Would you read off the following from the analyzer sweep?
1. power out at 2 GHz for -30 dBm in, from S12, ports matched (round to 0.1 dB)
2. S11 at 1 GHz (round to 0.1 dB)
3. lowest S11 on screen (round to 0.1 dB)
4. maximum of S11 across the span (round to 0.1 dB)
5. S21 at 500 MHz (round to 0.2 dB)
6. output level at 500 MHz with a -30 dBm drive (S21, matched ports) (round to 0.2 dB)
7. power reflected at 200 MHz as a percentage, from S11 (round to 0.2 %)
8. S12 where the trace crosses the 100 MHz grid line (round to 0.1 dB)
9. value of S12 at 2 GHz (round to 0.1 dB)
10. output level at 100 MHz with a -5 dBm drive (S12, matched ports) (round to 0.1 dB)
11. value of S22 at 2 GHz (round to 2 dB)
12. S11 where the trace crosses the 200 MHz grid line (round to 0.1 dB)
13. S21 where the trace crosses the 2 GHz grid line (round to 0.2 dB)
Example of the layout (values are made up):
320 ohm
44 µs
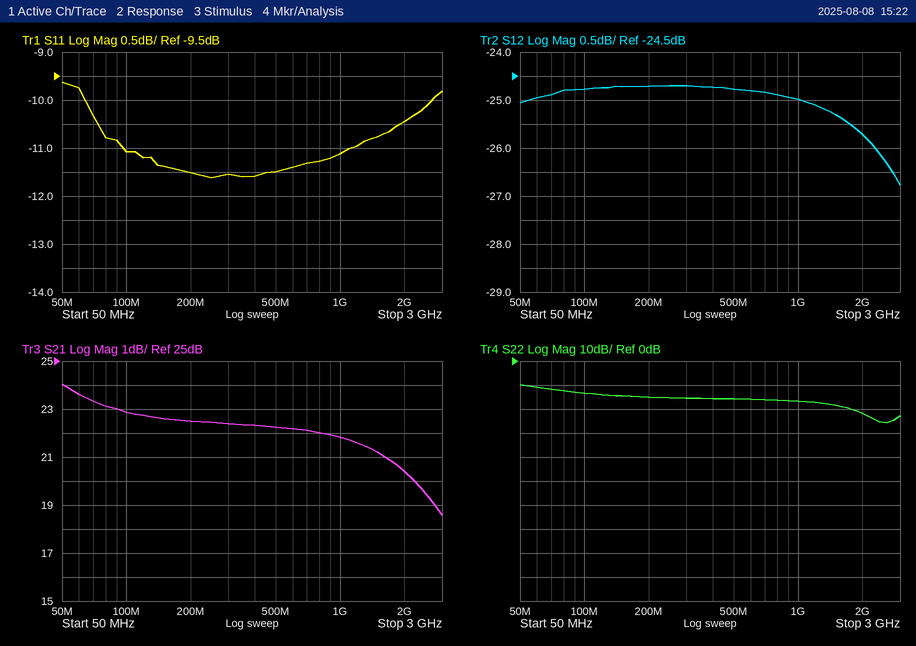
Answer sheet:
-55.7 dBm
-11.1 dB
-11.6 dB
-9.6 dB
22.2 dB
-7.8 dBm
7.0 %
-24.8 dB
-25.7 dB
-29.8 dBm
-22 dB
-11.5 dB
20.4 dB
